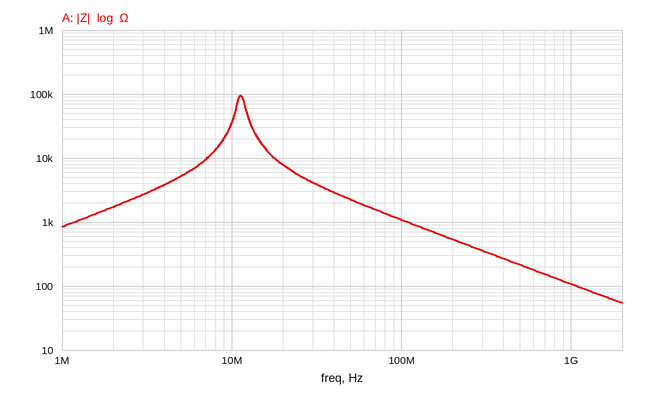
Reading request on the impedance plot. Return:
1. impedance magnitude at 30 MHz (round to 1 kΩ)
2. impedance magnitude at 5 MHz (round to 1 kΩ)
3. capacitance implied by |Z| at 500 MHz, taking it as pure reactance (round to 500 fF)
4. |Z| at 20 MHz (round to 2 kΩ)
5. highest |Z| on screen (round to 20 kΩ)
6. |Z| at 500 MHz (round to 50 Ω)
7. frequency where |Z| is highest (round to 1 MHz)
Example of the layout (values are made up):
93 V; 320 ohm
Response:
4 kΩ; 5 kΩ; 1.5 pF; 8 kΩ; 100 kΩ; 200 Ω; 11 MHz
